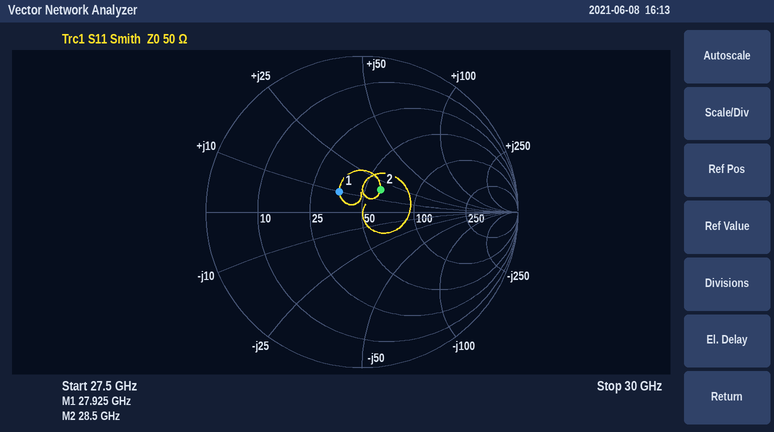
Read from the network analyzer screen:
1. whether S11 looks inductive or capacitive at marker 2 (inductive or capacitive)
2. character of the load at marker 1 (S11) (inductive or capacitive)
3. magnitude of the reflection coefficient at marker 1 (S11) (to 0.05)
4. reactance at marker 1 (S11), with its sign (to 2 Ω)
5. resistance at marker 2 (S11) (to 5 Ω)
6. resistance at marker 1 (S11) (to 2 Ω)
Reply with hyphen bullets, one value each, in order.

- inductive
- inductive
- 0.20
- +10 Ω
- 60 Ω
- 36 Ω
